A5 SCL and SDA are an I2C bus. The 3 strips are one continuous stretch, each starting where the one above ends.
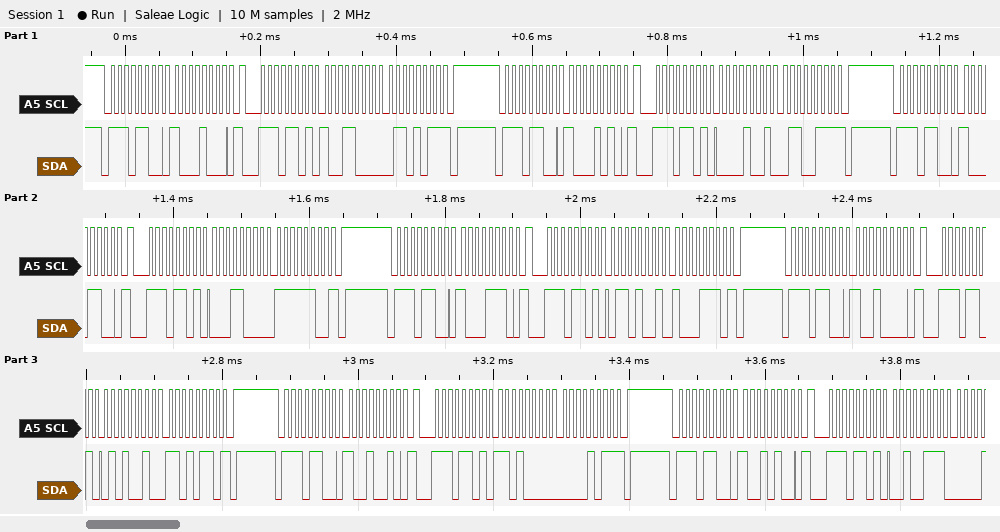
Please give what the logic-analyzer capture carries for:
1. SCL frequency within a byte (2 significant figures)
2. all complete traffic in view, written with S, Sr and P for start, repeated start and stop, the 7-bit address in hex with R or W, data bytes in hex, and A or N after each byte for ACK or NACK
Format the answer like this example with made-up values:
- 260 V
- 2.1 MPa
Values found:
- 100 kHz
- S 76W A 88 A Sr 76R A 98 A 6B N P S 76W A 8A A Sr 76R A 09 A 67 N P S 76W A 8C A Sr 76R A 18 A FC N P S 76W A 8E A Sr 76R A 69 A 8E N P S 76W A 90 A Sr 76R A 52 A D6 N P S 76W A 92 A Sr 76R A D0 A 0B N P S 76W A 94 A Sr 76R A 27 A
